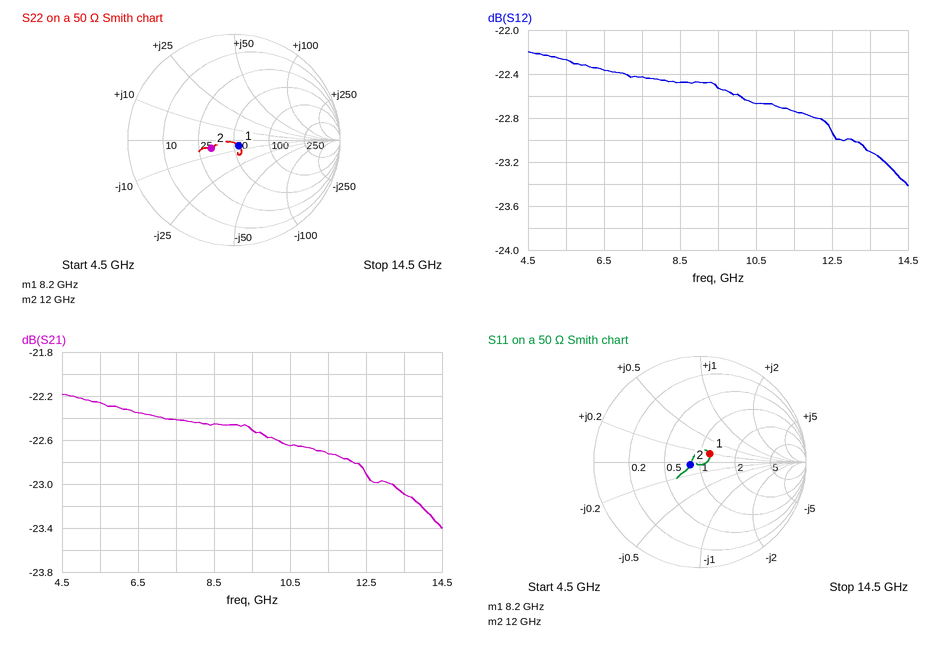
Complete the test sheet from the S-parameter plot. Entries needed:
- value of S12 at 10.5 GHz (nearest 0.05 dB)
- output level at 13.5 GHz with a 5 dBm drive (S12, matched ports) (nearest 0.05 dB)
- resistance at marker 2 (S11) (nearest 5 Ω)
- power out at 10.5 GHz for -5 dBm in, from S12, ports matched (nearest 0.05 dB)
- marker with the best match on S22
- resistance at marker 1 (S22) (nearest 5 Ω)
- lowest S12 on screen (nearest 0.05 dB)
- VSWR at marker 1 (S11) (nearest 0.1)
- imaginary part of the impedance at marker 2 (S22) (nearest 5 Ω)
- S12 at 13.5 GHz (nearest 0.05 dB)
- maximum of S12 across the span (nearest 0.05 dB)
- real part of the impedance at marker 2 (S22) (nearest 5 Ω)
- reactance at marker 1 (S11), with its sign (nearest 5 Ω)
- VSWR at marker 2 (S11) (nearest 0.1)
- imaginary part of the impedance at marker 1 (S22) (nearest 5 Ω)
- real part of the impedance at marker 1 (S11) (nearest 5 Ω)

-22.65 dB
-18.10 dBm
40 Ω
-27.65 dBm
marker 1
55 Ω
-23.40 dB
1.3
-5 Ω
-23.10 dB
-22.20 dB
30 Ω
+10 Ω
1.2
-5 Ω
60 Ω
